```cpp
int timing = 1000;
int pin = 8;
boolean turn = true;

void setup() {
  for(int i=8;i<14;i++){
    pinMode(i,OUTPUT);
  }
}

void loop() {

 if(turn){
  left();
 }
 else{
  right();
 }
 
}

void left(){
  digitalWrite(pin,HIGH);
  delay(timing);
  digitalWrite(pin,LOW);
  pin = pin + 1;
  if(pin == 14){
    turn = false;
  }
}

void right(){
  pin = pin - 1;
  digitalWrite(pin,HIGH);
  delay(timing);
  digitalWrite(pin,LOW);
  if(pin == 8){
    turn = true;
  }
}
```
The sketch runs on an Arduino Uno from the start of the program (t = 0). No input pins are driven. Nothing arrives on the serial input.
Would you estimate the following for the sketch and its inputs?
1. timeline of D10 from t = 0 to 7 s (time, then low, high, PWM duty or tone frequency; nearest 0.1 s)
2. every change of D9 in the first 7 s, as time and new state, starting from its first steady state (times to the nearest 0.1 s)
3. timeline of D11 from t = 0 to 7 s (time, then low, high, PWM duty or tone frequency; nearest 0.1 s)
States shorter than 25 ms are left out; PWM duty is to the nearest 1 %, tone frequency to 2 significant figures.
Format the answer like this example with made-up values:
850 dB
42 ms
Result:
0 s low; 2 s high; 3 s low
0 s low; 1 s high; 2 s low
0 s low; 3 s high; 4 s low
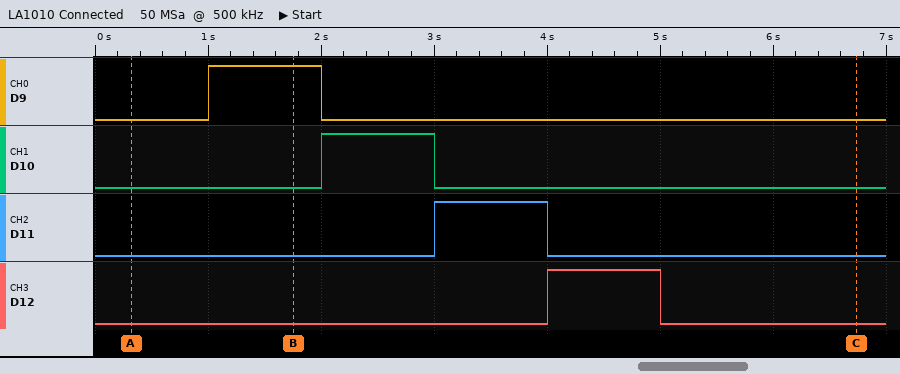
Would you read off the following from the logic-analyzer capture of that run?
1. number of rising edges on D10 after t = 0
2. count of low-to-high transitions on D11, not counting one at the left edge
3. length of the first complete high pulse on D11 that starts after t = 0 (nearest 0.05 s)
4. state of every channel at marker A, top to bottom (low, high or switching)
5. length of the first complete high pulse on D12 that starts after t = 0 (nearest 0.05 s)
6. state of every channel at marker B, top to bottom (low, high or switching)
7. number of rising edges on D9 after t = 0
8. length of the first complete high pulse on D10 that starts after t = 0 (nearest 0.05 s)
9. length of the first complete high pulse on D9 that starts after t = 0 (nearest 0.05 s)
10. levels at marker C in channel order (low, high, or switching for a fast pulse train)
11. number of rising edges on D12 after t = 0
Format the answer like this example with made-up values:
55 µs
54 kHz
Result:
1
1
1.00 s
D9 low, D10 low, D11 low, D12 low
1.00 s
D9 high, D10 low, D11 low, D12 low
1
1.00 s
1.00 s
D9 low, D10 low, D11 low, D12 low
1
